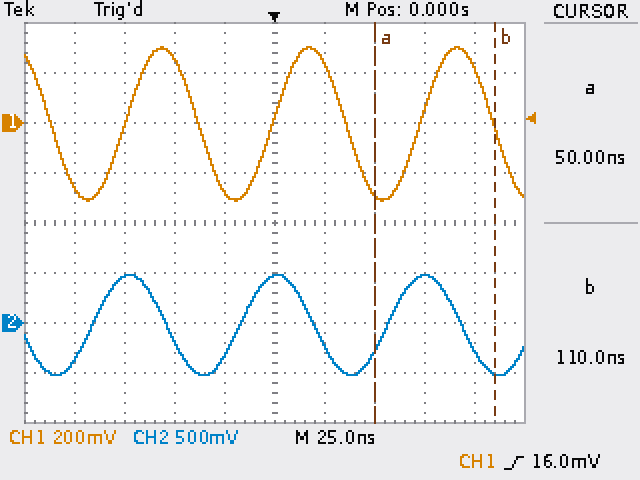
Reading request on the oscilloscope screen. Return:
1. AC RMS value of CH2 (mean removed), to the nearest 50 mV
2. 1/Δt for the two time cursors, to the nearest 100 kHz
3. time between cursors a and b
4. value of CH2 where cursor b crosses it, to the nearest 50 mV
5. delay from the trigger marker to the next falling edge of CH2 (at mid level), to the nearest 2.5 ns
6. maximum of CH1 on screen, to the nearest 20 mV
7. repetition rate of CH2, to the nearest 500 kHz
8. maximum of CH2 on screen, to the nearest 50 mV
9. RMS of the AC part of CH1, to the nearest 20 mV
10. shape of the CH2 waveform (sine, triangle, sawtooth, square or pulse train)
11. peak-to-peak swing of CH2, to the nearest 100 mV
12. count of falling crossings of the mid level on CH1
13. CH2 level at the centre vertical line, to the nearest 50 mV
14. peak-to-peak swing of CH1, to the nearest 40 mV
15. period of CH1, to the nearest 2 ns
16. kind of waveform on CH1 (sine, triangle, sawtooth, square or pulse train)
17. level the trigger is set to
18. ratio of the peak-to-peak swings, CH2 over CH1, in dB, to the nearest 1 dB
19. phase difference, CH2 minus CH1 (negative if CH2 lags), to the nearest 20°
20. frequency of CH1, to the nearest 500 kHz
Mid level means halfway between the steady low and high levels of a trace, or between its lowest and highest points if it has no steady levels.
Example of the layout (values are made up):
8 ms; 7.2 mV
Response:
350 mV; 16.7 MHz; 60.0 ns; -500 mV; 20.0 ns; 300 mV; 13.5 MHz; 500 mV; 220 mV; sine; 1.00 V; 4; 450 mV; 600 mV; 74 ns; sine; 16.0 mV; 4 dB; +80°; 13.5 MHz
